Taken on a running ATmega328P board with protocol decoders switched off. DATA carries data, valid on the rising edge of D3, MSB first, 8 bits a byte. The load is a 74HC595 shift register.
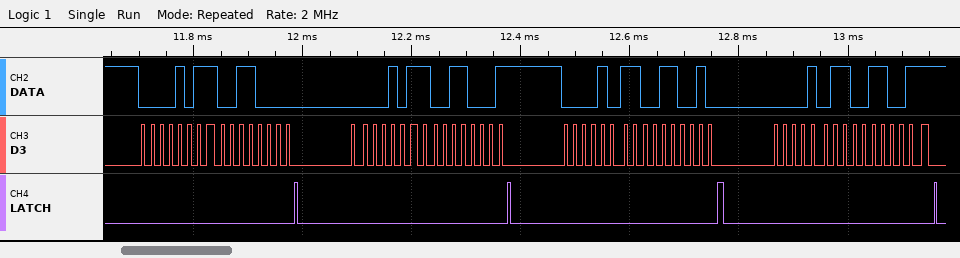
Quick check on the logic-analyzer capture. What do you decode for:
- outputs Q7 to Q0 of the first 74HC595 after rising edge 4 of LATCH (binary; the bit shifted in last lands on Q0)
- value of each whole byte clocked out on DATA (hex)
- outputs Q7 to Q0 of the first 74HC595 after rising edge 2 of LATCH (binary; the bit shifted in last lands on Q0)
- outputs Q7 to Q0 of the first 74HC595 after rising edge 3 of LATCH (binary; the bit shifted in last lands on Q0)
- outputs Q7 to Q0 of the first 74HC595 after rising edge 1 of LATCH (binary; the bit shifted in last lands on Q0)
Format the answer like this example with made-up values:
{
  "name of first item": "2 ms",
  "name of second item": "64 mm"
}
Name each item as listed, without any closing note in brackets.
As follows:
{
  "outputs Q7 to Q0 of the first 74HC595 after rising edge 4 of LATCH": "00110011",
  "value of each whole byte clocked out on DATA": "0B 30 0B 31 0B 32 0B 33",
  "outputs Q7 to Q0 of the first 74HC595 after rising edge 2 of LATCH": "00110001",
  "outputs Q7 to Q0 of the first 74HC595 after rising edge 3 of LATCH": "00110010",
  "outputs Q7 to Q0 of the first 74HC595 after rising edge 1 of LATCH": "00110000"
}
